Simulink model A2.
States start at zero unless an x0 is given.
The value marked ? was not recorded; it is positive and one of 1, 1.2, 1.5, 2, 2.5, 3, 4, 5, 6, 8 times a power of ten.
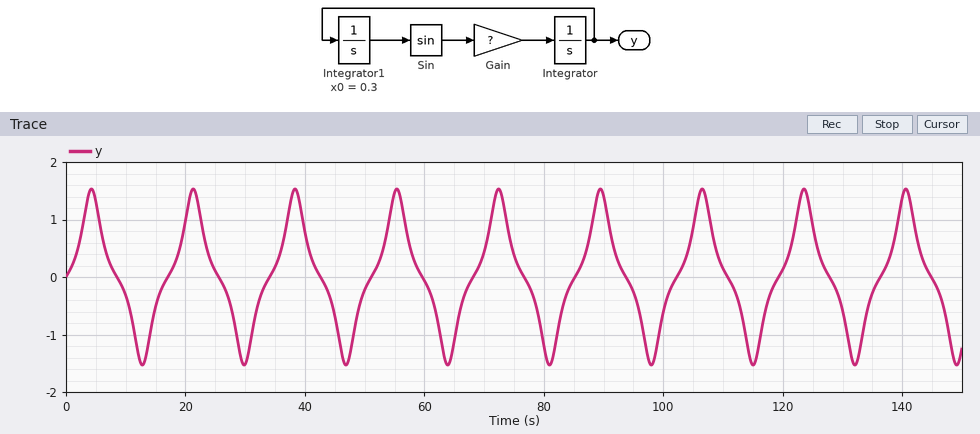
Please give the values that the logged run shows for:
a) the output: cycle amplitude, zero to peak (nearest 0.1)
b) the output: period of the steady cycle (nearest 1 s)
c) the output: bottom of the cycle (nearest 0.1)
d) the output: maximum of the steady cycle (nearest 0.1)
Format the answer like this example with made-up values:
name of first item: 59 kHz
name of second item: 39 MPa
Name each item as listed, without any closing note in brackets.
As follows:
the output: cycle amplitude, zero to peak: 1.5
the output: period of the steady cycle: 17 s
the output: bottom of the cycle: -1.5
the output: maximum of the steady cycle: 1.5
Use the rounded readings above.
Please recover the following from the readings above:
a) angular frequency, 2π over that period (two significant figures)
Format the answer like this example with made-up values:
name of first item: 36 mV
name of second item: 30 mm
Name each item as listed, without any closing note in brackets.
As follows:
angular frequency, 2π over that period: 0.37 rad/s
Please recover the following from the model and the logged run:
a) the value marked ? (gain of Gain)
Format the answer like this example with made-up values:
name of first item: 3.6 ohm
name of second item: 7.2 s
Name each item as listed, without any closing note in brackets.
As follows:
the value marked ?: 0.6
